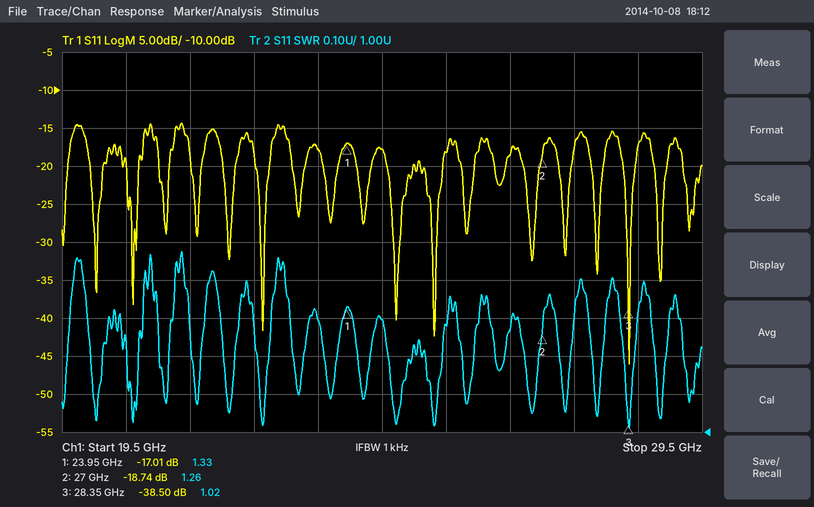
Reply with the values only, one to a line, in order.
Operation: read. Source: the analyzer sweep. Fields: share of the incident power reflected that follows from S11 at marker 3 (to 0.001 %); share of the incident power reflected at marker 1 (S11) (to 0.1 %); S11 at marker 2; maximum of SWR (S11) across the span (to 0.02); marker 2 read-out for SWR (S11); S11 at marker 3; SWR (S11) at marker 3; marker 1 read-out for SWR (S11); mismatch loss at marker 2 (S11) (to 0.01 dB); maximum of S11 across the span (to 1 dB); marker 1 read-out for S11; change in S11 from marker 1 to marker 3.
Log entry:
0.014 %
2.0 %
-18.74 dB
1.48
1.26
-38.50 dB
1.02
1.33
0.06 dB
-14 dB
-17.01 dB
-21.49 dB
